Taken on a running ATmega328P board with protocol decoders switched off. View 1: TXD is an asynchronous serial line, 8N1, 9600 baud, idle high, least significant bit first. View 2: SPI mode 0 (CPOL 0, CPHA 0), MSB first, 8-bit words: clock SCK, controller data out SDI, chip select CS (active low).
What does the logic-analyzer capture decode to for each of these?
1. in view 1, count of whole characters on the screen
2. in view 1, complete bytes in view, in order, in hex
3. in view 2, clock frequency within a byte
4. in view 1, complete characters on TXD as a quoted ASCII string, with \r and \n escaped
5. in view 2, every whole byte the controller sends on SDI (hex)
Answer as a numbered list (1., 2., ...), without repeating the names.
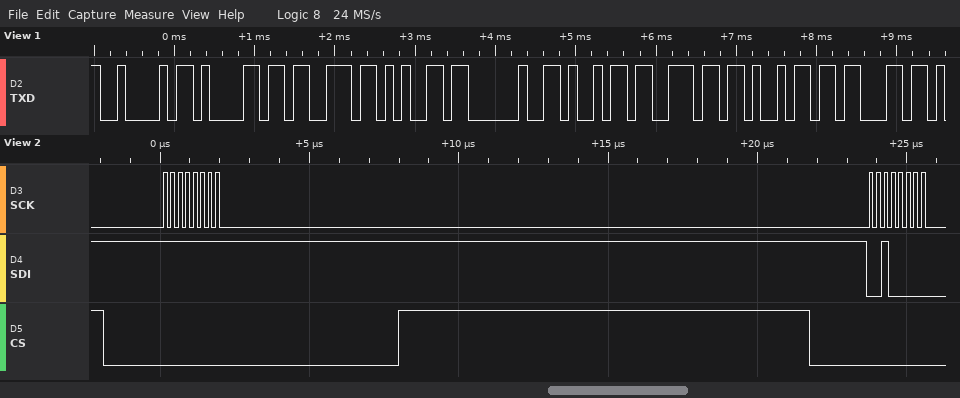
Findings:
1. 9
2. 42 61 73 65 20 69 6E 69 63
3. 4 MHz
4. "Base inic"
5. 0xFF 0x20
